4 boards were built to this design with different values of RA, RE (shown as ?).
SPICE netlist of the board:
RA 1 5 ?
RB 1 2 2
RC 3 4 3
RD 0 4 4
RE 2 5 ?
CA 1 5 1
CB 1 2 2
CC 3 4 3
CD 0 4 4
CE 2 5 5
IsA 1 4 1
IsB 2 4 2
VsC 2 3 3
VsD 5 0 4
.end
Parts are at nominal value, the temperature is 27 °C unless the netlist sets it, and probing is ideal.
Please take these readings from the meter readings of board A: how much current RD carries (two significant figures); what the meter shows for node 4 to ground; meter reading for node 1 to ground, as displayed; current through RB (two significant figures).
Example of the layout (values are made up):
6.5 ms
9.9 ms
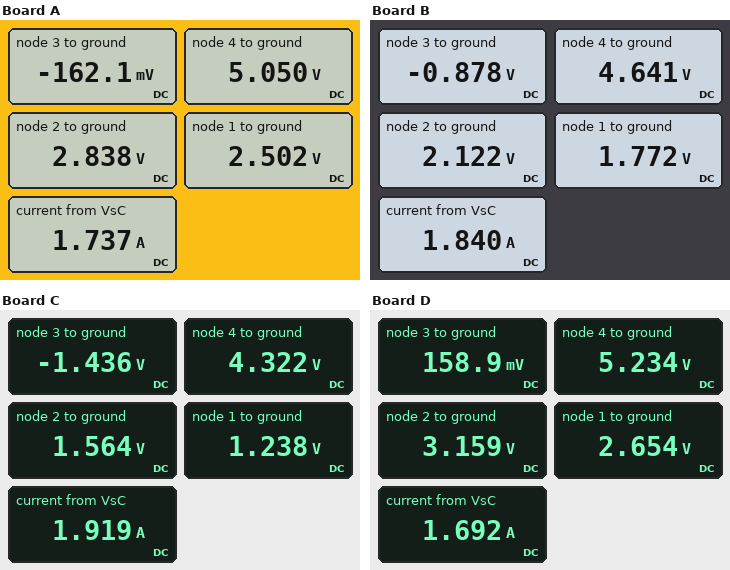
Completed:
1.3 A
5.050 V
2.502 V
170 mA
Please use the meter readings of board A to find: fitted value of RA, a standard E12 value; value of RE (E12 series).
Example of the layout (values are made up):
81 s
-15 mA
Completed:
1.8 Ω
2.7 Ω
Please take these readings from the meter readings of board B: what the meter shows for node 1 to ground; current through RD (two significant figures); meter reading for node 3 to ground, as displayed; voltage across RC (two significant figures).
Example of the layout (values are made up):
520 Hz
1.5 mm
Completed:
1.772 V
1.2 A
-0.878 V
5.5 V
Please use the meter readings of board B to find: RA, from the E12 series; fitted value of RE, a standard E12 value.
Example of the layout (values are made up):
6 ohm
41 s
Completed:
2.7 Ω
5.6 Ω
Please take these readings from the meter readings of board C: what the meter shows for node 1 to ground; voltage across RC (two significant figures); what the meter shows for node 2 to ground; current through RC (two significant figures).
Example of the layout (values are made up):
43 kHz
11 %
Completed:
1.238 V
5.8 V
1.564 V
1.9 A
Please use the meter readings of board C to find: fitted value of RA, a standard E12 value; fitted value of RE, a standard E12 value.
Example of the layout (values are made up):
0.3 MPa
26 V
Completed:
3.3 Ω
10 Ω
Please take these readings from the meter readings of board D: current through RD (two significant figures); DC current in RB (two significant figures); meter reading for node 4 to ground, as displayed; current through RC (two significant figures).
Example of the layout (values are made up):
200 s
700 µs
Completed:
1.3 A
250 mA
5.234 V
1.7 A
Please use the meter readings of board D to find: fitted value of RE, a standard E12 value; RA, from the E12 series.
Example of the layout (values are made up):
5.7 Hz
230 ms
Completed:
1.5 Ω
1.8 Ω
